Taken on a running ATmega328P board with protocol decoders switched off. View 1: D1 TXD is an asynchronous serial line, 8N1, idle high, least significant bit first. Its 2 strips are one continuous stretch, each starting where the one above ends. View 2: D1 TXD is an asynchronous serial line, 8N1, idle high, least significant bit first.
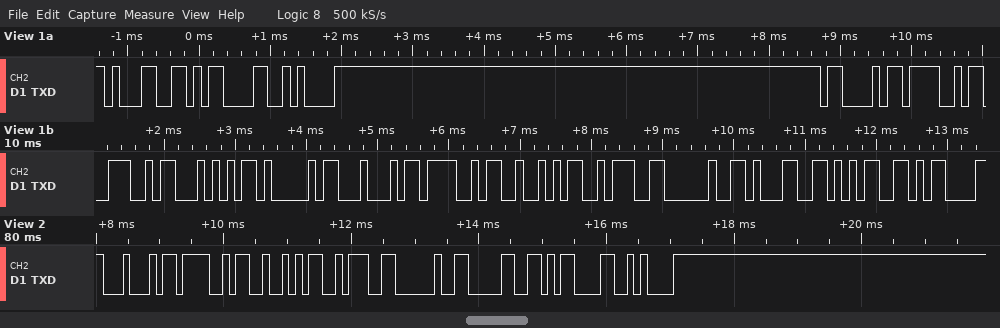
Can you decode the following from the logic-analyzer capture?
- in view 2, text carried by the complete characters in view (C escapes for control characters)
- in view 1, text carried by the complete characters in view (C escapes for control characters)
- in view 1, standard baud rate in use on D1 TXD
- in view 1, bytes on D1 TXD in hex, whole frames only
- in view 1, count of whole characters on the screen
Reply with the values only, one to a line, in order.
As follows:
"DOR: 0\r\n"
"1\r\nCONTADOR: 15\r"
9600 baud
31 0D 0A 43 4F 4E 54 41 44 4F 52 3A 20 31 35 0D
16
